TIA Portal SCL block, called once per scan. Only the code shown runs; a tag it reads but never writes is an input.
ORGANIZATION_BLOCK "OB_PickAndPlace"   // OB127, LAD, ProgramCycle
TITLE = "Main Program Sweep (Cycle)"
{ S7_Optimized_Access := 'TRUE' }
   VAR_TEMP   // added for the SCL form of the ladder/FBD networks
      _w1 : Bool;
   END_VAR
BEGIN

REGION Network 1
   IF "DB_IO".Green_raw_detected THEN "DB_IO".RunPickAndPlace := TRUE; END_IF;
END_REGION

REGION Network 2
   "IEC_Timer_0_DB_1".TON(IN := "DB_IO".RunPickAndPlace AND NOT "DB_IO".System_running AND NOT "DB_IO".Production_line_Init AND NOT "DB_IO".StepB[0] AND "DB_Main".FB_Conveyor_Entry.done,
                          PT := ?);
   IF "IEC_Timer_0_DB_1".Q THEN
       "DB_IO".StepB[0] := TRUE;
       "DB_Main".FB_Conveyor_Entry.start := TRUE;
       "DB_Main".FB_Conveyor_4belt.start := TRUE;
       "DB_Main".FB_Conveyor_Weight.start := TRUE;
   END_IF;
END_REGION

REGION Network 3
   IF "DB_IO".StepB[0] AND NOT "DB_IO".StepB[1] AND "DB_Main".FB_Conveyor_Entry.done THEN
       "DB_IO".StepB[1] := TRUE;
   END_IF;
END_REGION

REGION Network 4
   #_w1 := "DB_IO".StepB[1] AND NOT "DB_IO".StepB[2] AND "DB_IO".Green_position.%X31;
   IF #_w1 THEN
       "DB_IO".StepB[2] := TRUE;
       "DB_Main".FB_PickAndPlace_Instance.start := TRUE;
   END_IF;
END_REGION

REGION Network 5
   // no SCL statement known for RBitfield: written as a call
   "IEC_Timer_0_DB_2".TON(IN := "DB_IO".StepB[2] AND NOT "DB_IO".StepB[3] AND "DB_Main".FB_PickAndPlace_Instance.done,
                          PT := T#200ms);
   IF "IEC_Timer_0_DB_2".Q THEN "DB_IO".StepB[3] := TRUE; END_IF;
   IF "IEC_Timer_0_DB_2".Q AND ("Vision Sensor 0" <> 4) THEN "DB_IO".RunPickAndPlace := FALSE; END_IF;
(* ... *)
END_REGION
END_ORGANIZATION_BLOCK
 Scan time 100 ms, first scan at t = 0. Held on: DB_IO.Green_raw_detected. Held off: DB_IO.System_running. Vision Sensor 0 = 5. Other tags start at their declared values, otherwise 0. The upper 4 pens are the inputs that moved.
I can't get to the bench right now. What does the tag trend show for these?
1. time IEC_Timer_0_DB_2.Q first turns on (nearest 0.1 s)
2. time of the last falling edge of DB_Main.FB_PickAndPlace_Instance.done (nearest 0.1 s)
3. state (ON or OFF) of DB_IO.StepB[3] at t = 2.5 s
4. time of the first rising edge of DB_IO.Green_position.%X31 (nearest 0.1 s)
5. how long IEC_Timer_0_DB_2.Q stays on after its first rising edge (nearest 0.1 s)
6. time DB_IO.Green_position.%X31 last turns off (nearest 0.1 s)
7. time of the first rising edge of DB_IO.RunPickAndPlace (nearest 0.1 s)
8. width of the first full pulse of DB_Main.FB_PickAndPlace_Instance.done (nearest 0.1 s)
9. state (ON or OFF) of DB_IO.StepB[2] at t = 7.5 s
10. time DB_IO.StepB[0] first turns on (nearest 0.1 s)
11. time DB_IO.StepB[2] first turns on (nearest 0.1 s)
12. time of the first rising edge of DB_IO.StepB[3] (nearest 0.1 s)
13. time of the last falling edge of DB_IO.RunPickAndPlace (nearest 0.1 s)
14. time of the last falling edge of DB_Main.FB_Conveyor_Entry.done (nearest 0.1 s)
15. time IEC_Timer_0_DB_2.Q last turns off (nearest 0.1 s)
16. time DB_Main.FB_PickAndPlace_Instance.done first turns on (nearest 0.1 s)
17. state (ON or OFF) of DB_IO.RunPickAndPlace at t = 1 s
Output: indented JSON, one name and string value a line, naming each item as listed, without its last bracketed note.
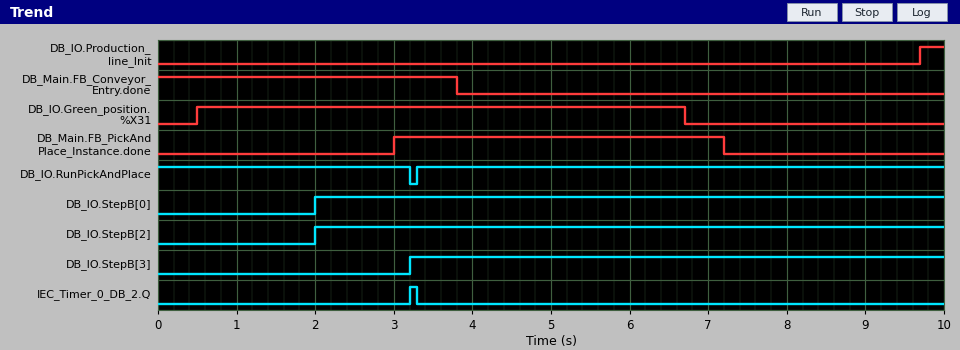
{
  "time IEC_Timer_0_DB_2.Q first turns on": "3.2 s",
  "time of the last falling edge of DB_Main.FB_PickAndPlace_Instance.done": "7.2 s",
  "state (ON or OFF) of DB_IO.StepB[3] at t = 2.5 s": "OFF",
  "time of the first rising edge of DB_IO.Green_position.%X31": "0.5 s",
  "how long IEC_Timer_0_DB_2.Q stays on after its first rising edge": "0.1 s",
  "time DB_IO.Green_position.%X31 last turns off": "6.7 s",
  "time of the first rising edge of DB_IO.RunPickAndPlace": "3.3 s",
  "width of the first full pulse of DB_Main.FB_PickAndPlace_Instance.done": "4.2 s",
  "state (ON or OFF) of DB_IO.StepB[2] at t = 7.5 s": "ON",
  "time DB_IO.StepB[0] first turns on": "2.0 s",
  "time DB_IO.StepB[2] first turns on": "2.0 s",
  "time of the first rising edge of DB_IO.StepB[3]": "3.2 s",
  "time of the last falling edge of DB_IO.RunPickAndPlace": "3.2 s",
  "time of the last falling edge of DB_Main.FB_Conveyor_Entry.done": "3.8 s",
  "time IEC_Timer_0_DB_2.Q last turns off": "3.3 s",
  "time DB_Main.FB_PickAndPlace_Instance.done first turns on": "3.0 s",
  "state (ON or OFF) of DB_IO.RunPickAndPlace at t = 1 s": "ON"
}
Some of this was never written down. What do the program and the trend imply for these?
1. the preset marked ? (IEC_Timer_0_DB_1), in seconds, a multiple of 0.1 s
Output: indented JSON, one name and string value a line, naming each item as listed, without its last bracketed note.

{
  "the preset marked ? (IEC_Timer_0_DB_1), in seconds, a multiple of 0.1 s": "2.0 s"
}
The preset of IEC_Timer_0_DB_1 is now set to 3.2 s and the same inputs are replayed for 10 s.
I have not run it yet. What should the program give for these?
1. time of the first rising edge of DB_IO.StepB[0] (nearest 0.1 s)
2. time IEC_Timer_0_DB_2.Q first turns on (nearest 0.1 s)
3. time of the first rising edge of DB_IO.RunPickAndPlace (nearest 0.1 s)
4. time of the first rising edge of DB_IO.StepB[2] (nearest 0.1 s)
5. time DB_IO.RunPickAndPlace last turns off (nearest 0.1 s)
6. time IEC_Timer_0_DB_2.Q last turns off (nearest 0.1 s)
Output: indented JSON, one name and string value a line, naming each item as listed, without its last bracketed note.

{
  "time of the first rising edge of DB_IO.StepB[0]": "3.2 s",
  "time IEC_Timer_0_DB_2.Q first turns on": "3.4 s",
  "time of the first rising edge of DB_IO.RunPickAndPlace": "3.5 s",
  "time of the first rising edge of DB_IO.StepB[2]": "3.2 s",
  "time DB_IO.RunPickAndPlace last turns off": "3.4 s",
  "time IEC_Timer_0_DB_2.Q last turns off": "3.5 s"
}
